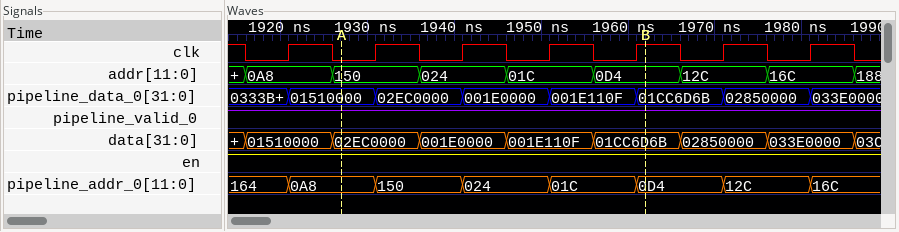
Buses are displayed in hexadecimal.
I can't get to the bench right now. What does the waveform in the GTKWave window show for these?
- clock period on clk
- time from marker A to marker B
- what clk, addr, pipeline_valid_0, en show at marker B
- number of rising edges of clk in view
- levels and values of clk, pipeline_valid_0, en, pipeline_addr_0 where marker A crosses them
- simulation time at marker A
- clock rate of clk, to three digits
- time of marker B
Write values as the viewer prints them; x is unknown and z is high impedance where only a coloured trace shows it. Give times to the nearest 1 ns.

10 ns
35 ns
clk=1, addr=0D4, pipeline_valid_0=1, en=1
7
clk=0, pipeline_valid_0=1, en=1, pipeline_addr_0=0A8
1927 ns
100 MHz
1962 ns
